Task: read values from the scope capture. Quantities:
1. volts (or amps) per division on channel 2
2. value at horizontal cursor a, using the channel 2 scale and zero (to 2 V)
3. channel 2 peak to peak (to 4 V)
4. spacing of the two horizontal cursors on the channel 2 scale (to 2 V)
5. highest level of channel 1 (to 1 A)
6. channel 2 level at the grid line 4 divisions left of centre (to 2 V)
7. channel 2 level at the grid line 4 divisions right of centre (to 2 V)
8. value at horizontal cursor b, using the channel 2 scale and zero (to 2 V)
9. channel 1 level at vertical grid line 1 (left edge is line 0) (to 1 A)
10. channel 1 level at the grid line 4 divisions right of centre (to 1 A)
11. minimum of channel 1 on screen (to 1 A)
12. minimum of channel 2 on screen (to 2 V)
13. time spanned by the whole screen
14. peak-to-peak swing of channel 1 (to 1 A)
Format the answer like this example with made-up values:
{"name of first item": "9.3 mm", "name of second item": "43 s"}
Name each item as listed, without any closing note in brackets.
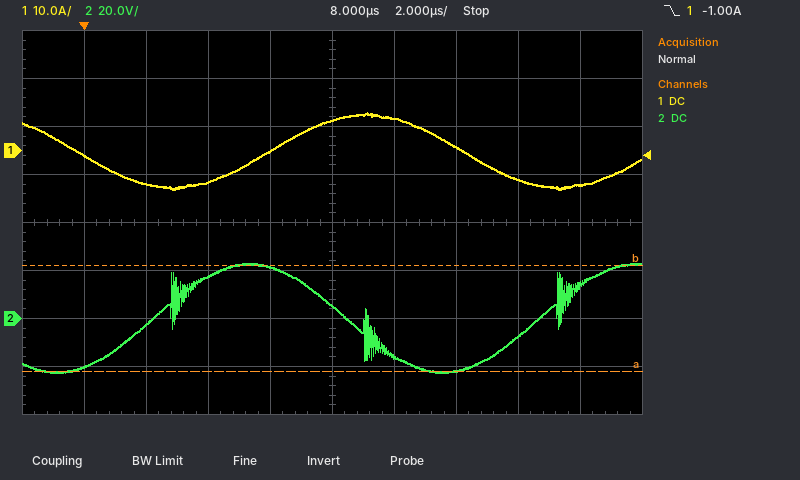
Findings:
{"volts (or amps) per division on channel 2": "20 V", "value at horizontal cursor a, using the channel 2 scale and zero": "-22 V", "channel 2 peak to peak": "44 V", "spacing of the two horizontal cursors on the channel 2 scale": "44 V", "highest level of channel 1": "8 A", "channel 2 level at the grid line 4 divisions left of centre": "-20 V", "channel 2 level at the grid line 4 divisions right of centre": "14 V", "value at horizontal cursor b, using the channel 2 scale and zero": "22 V", "channel 1 level at vertical grid line 1 (left edge is line 0)": "-1 A", "channel 1 level at the grid line 4 divisions right of centre": "-7 A", "minimum of channel 1 on screen": "-8 A", "minimum of channel 2 on screen": "-22 V", "time spanned by the whole screen": "20 µs", "peak-to-peak swing of channel 1": "16 A"}
